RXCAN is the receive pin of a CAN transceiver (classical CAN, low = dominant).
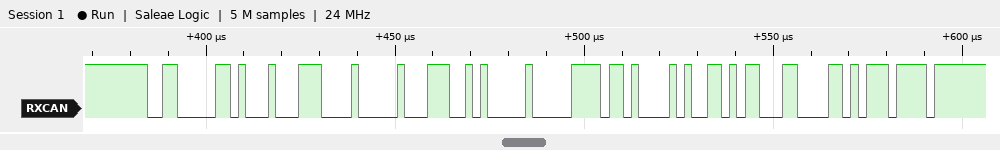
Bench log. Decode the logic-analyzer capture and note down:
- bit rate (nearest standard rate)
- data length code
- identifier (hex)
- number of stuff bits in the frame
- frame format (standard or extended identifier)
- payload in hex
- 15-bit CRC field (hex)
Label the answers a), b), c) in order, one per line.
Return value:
a) 500 kbit/s
b) 8
c) 0x305
d) 4
e) standard
f) E1 00 E5 00 3B 42 9A C6
g) 0x0D77
